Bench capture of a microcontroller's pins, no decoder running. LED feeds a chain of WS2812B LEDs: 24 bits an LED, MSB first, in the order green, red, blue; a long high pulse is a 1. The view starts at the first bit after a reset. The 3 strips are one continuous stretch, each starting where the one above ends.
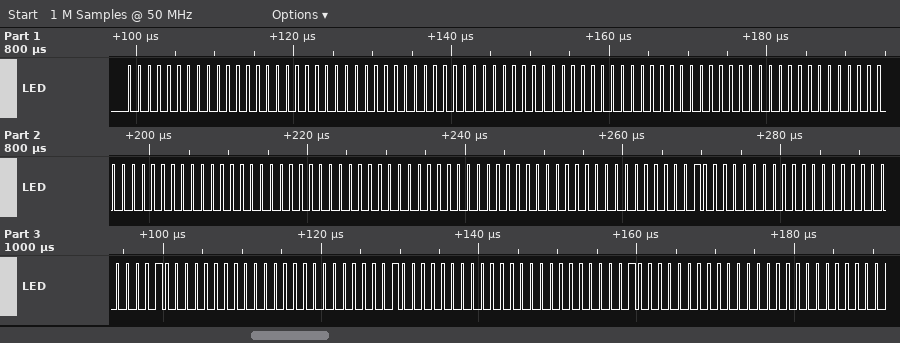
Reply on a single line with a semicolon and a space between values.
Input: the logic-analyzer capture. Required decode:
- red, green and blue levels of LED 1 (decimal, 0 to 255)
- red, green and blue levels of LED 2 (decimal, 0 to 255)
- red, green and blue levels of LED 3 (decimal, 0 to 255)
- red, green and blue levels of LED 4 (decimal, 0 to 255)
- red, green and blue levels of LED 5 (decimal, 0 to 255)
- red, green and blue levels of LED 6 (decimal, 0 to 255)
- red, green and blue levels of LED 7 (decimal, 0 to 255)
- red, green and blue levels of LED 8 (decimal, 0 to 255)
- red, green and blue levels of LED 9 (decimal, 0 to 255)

0, 0, 0; 0, 0, 0; 0, 0, 0; 0, 0, 0; 0, 0, 0; 0, 0, 128; 0, 0, 128; 0, 0, 128; 0, 0, 128
